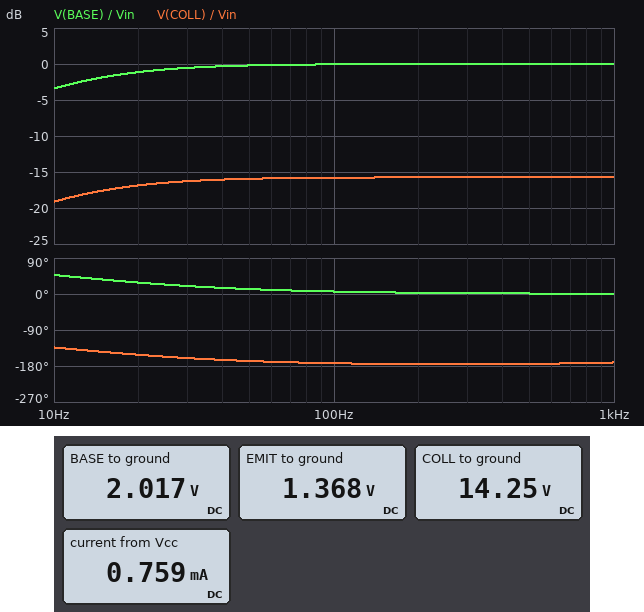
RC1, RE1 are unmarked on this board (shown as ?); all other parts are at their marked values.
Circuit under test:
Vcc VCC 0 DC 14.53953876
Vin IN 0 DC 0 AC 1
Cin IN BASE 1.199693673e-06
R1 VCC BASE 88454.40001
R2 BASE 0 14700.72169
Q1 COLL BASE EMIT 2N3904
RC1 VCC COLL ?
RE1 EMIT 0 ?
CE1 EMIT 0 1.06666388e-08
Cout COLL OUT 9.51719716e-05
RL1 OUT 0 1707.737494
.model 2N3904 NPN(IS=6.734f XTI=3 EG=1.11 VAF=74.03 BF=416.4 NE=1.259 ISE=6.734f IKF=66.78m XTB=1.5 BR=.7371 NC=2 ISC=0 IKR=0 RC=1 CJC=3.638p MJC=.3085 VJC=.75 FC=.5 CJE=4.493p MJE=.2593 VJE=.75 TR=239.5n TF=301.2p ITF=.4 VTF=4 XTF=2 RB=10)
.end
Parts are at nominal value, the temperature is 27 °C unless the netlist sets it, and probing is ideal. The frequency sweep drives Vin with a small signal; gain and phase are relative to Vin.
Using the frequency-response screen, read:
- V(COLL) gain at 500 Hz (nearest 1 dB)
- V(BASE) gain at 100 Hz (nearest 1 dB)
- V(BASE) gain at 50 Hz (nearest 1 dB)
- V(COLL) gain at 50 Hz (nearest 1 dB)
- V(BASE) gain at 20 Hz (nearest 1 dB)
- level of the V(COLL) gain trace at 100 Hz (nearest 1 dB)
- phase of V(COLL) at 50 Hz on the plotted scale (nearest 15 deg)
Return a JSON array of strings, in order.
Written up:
["-16 dB", "0 dB", "0 dB", "-16 dB", "-1 dB", "-16 dB", "-165 deg"]
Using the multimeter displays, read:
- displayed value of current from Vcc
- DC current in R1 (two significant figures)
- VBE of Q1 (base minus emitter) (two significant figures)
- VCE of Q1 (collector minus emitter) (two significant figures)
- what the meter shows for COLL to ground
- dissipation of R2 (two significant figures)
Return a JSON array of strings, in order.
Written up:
["0.759 mA", "140 µA", "650 mV", "13 V", "14.25 V", "280 µW"]
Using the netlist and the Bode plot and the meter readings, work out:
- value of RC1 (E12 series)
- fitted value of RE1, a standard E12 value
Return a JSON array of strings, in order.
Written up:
["470 Ω", "2.2 kΩ"]
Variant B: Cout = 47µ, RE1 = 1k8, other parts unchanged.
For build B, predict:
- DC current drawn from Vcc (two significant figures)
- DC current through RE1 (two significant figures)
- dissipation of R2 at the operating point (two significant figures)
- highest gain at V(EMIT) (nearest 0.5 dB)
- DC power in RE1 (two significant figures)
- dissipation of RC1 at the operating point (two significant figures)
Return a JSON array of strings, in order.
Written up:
["890 µA", "750 µA", "270 µW", "0 dB", "1.0 mW", "260 µW"]
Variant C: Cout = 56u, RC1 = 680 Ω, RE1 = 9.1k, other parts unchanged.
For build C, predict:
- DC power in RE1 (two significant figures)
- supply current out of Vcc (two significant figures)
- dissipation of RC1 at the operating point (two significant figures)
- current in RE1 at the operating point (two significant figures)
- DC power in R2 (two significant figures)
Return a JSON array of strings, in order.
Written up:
["230 µW", "300 µA", "17 µW", "160 µA", "290 µW"]
